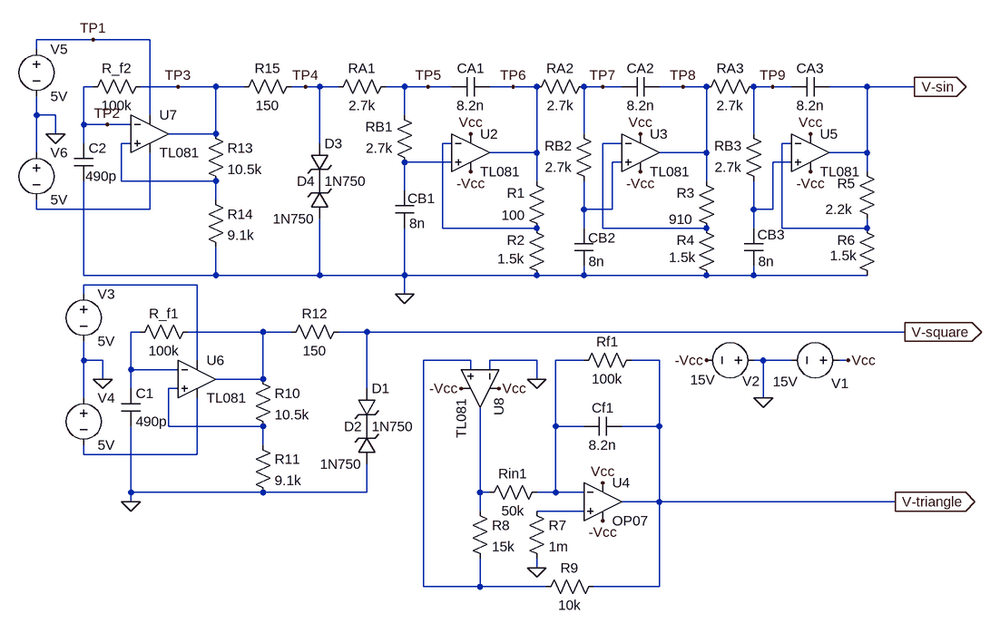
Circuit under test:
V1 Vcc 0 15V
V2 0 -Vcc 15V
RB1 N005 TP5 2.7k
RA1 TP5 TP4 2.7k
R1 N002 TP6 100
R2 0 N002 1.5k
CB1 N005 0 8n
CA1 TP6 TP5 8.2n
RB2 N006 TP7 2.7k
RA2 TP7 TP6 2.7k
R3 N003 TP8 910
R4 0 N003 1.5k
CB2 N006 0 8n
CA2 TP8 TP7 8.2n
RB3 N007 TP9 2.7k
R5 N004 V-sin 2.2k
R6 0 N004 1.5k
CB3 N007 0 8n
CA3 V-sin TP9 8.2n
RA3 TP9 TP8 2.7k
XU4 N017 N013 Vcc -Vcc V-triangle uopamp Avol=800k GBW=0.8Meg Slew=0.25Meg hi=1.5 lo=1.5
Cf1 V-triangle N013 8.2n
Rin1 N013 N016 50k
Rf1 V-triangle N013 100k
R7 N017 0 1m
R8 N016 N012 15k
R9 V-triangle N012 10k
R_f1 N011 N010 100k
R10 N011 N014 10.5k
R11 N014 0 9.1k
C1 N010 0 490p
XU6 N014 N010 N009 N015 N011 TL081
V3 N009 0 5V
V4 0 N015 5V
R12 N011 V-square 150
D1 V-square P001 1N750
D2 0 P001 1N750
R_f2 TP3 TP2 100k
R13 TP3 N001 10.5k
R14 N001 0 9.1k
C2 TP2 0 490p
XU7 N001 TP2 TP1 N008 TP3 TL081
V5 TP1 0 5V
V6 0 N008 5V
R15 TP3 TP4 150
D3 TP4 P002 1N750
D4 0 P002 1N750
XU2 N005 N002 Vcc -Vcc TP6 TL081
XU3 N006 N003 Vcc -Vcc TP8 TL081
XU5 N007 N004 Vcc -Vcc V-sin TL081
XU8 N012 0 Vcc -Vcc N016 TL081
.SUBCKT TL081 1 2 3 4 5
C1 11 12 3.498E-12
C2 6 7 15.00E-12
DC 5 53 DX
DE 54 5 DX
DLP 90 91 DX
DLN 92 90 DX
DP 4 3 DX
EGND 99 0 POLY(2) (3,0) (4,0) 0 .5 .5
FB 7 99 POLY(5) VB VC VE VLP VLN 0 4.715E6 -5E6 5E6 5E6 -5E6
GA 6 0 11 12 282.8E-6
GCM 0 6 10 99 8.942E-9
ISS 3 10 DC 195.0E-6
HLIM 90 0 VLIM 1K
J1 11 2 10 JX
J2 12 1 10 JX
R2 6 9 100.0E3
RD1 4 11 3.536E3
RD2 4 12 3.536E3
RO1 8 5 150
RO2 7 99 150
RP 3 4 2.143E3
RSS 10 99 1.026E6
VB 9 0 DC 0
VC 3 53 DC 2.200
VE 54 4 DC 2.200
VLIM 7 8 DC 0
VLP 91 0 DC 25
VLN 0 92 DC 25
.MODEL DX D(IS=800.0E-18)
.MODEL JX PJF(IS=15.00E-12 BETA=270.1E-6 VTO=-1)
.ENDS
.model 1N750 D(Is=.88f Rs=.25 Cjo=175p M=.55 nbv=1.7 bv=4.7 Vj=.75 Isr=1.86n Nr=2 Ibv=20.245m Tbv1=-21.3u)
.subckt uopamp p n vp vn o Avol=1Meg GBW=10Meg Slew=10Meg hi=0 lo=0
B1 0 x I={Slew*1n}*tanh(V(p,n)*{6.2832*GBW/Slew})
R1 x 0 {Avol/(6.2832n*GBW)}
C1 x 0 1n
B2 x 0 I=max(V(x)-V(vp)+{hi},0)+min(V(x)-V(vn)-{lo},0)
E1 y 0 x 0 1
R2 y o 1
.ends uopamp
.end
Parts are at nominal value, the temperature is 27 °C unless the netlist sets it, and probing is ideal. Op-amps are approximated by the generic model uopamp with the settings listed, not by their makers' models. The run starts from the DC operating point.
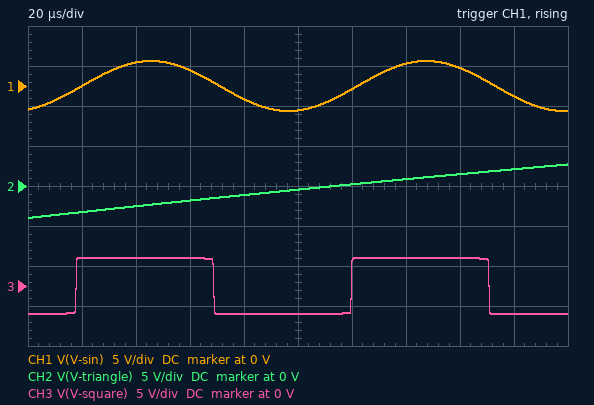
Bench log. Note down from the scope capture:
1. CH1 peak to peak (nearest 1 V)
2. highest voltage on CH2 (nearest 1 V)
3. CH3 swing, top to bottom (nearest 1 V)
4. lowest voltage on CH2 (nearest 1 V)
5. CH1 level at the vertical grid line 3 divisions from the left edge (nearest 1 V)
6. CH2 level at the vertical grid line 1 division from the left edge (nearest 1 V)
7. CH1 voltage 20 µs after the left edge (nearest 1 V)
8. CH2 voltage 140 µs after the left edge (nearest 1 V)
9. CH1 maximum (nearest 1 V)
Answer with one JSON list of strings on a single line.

["6 V", "3 V", "7 V", "-4 V", "2 V", "-3 V", "0 V", "1 V", "3 V"]
